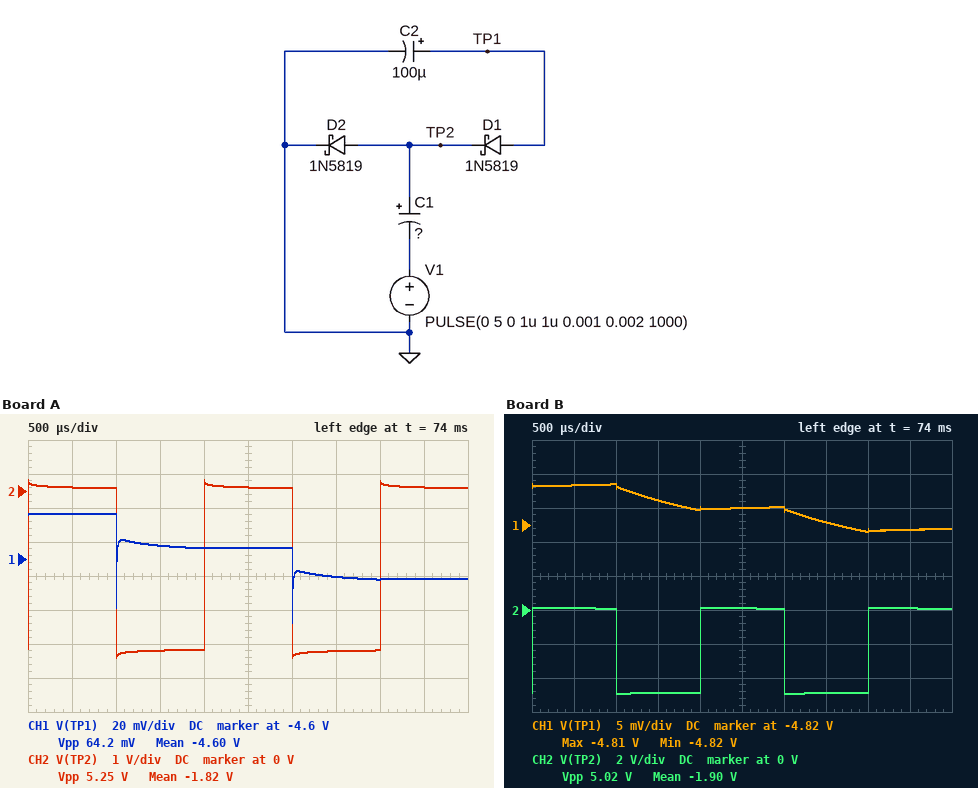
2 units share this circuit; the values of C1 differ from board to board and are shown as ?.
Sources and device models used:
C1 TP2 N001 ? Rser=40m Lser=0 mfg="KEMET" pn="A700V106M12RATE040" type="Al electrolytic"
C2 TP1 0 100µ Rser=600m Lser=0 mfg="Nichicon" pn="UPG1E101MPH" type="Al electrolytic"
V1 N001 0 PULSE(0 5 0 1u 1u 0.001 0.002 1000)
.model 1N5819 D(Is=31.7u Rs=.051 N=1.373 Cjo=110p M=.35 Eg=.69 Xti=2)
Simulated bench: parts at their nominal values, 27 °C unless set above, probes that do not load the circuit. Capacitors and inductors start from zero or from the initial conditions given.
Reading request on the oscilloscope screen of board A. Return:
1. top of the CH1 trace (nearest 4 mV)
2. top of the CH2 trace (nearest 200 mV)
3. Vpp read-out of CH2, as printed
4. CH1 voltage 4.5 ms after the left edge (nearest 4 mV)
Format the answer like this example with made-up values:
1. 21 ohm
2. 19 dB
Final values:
1. -4.572 V
2. 400 mV
3. 5.25 V
4. -4.612 V
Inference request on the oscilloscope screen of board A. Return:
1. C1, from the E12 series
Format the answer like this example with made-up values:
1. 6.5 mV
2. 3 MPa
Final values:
1. 8.2 µF
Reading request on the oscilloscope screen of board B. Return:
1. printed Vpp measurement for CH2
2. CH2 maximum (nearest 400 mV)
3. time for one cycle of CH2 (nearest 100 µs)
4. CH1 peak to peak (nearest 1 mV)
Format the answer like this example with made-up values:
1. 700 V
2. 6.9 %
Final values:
1. 5.02 V
2. 0 V
3. 2.0 ms
4. 7 mV
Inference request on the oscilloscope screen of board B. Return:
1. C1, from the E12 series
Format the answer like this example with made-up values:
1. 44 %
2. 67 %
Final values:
1. 22 µF
